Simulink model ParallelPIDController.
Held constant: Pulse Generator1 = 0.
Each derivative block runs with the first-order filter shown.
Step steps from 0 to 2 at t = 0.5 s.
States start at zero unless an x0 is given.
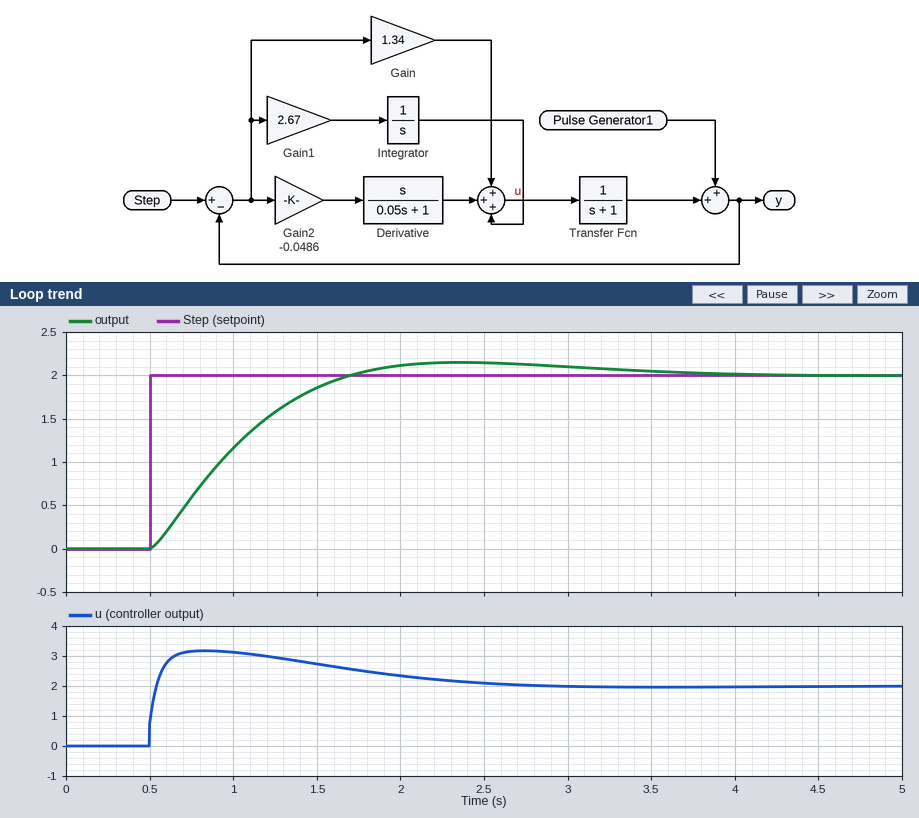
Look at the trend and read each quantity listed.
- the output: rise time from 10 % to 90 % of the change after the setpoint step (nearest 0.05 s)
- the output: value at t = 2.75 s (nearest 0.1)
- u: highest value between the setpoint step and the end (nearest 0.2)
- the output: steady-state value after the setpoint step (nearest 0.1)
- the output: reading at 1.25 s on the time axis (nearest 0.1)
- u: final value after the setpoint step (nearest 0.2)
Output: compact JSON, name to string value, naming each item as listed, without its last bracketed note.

{"the output: rise time from 10 % to 90 % of the change after the setpoint step": "0.85 s", "the output: value at t = 2.75 s": "2.1", "u: highest value between the setpoint step and the end": "3.2", "the output: steady-state value after the setpoint step": "2.0", "the output: reading at 1.25 s on the time axis": "1.6", "u: final value after the setpoint step": "2.0"}
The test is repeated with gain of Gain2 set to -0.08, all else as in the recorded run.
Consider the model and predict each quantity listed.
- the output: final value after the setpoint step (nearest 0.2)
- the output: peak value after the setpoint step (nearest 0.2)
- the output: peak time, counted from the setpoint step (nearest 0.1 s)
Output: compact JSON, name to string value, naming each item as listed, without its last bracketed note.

{"the output: final value after the setpoint step": "2.0", "the output: peak value after the setpoint step": "2.2", "the output: peak time, counted from the setpoint step": "1.8 s"}
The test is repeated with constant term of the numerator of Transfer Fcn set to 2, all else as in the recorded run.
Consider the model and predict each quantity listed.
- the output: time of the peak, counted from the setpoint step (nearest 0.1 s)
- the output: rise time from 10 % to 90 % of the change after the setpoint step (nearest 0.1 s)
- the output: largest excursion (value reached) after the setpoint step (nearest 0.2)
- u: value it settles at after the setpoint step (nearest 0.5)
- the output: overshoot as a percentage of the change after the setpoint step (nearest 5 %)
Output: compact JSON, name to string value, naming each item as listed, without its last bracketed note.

{"the output: time of the peak, counted from the setpoint step": "1.1 s", "the output: rise time from 10 % to 90 % of the change after the setpoint step": "0.5 s", "the output: largest excursion (value reached) after the setpoint step": "2.2", "u: value it settles at after the setpoint step": "1.0", "the output: overshoot as a percentage of the change after the setpoint step": "10 %"}
